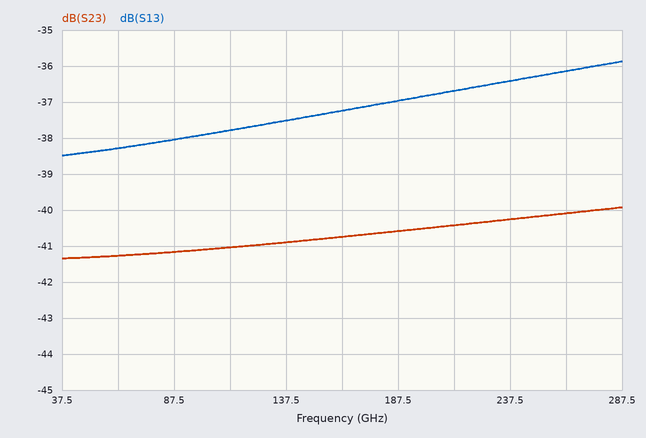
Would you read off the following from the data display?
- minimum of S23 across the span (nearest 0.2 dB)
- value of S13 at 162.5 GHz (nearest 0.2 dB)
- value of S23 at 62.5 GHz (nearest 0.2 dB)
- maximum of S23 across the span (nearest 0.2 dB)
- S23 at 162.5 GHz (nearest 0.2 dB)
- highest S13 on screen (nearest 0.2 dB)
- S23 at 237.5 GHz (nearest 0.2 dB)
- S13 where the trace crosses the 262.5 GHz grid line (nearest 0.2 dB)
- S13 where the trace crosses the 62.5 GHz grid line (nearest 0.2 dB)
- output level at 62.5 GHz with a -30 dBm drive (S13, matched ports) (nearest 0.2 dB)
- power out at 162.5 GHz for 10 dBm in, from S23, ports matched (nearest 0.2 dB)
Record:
-41.4 dB
-37.2 dB
-41.2 dB
-40.0 dB
-40.8 dB
-35.8 dB
-40.2 dB
-36.2 dB
-38.2 dB
-68.2 dBm
-30.8 dBm
